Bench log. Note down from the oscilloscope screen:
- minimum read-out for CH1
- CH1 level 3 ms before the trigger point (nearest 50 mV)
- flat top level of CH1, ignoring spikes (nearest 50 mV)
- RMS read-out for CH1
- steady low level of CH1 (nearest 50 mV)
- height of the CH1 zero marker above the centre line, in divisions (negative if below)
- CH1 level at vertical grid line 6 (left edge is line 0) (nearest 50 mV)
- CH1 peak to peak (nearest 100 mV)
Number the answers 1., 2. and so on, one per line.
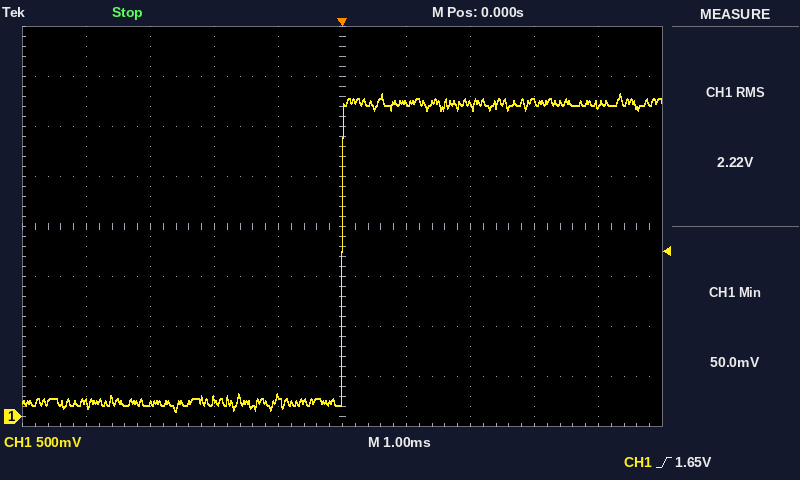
1. 50.0 mV
2. 150 mV
3. 3.15 V
4. 2.22 V
5. 150 mV
6. -3.8 div
7. 3.15 V
8. 3.20 V
